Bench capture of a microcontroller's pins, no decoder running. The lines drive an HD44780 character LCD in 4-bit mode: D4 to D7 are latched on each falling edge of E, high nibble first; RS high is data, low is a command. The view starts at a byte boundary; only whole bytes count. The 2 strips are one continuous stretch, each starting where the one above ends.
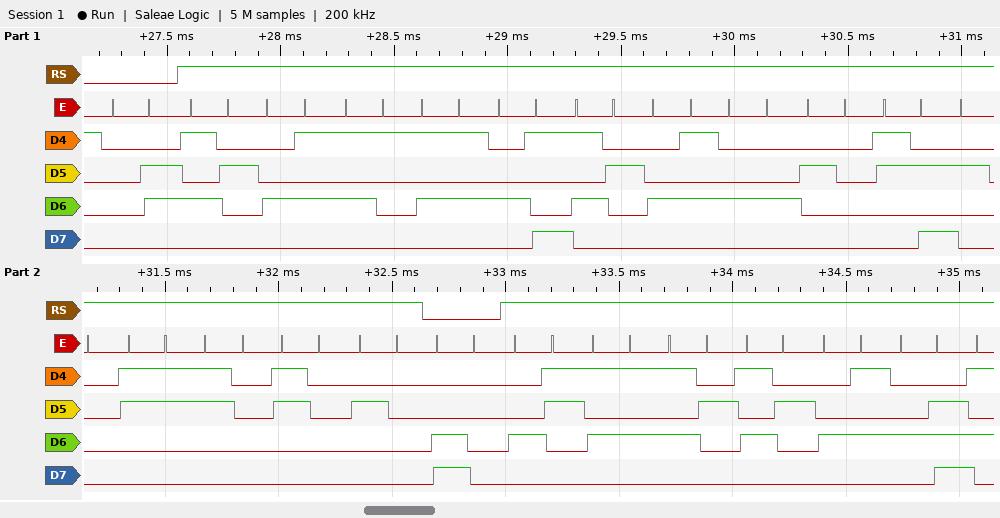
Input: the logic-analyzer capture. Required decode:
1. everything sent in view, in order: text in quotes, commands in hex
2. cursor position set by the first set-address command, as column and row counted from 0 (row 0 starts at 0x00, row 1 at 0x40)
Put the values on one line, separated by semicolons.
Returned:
0x06 "REQUIRED : 300 " 0xC0 "CURREN"; column 0, row 1
